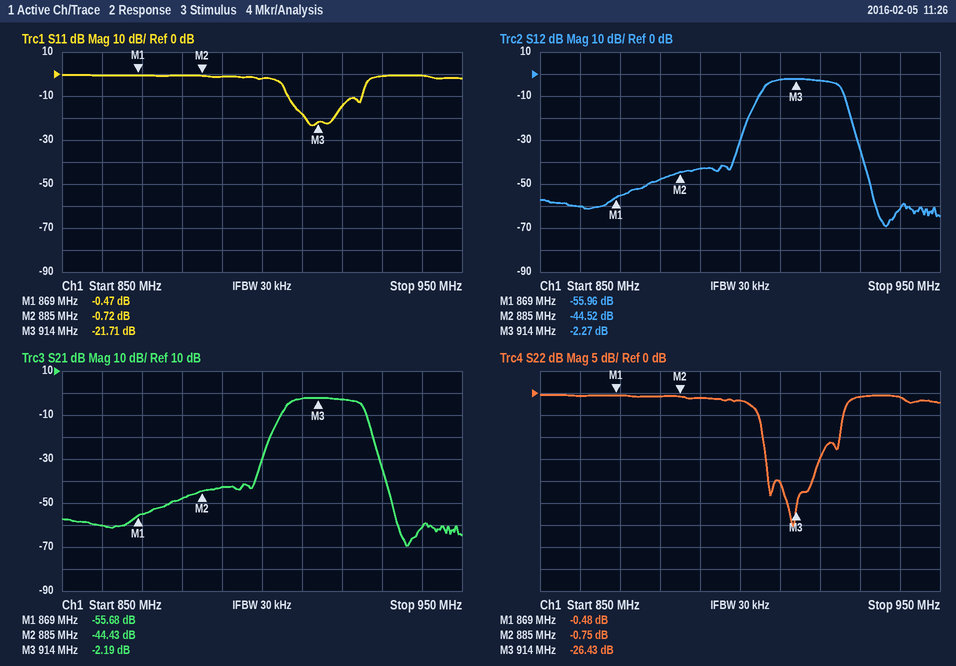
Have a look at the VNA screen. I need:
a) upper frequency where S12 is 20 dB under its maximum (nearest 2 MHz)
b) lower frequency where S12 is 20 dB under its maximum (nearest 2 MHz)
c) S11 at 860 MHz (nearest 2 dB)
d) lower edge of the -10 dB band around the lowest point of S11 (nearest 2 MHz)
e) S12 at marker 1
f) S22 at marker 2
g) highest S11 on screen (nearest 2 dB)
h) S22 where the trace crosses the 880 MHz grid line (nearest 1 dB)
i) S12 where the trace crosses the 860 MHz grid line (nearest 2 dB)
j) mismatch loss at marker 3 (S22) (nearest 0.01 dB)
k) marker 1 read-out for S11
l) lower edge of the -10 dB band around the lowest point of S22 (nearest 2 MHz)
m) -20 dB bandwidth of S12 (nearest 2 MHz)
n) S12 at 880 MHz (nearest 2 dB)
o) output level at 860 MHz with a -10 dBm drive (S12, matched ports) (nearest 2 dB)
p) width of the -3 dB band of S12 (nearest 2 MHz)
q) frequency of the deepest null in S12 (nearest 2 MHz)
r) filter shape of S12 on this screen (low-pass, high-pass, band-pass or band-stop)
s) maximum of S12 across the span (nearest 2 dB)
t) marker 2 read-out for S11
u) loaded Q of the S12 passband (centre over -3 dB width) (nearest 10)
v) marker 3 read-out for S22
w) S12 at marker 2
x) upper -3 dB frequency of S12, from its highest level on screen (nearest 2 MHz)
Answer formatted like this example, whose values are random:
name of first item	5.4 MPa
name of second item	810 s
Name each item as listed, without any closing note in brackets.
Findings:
upper frequency where S12 is 20 dB under its maximum	928 MHz
lower frequency where S12 is 20 dB under its maximum	902 MHz
S11 at 860 MHz	0 dB
lower edge of the -10 dB band around the lowest point of S11	906 MHz
S12 at marker 1	-55.96 dB
S22 at marker 2	-0.75 dB
highest S11 on screen	0 dB
S22 where the trace crosses the 880 MHz grid line	-1 dB
S12 where the trace crosses the 860 MHz grid line	-60 dB
mismatch loss at marker 3 (S22)	0.01 dB
marker 1 read-out for S11	-0.47 dB
lower edge of the -10 dB band around the lowest point of S22	906 MHz
-20 dB bandwidth of S12	26 MHz
S12 at 880 MHz	-48 dB
output level at 860 MHz with a -10 dBm drive (S12, matched ports)	-70 dBm
width of the -3 dB band of S12	18 MHz
frequency of the deepest null in S12	936 MHz
filter shape of S12 on this screen	band-pass
maximum of S12 across the span	-2 dB
marker 2 read-out for S11	-0.72 dB
loaded Q of the S12 passband (centre over -3 dB width)	50
marker 3 read-out for S22	-26.43 dB
S12 at marker 2	-44.52 dB
upper -3 dB frequency of S12, from its highest level on screen	924 MHz
